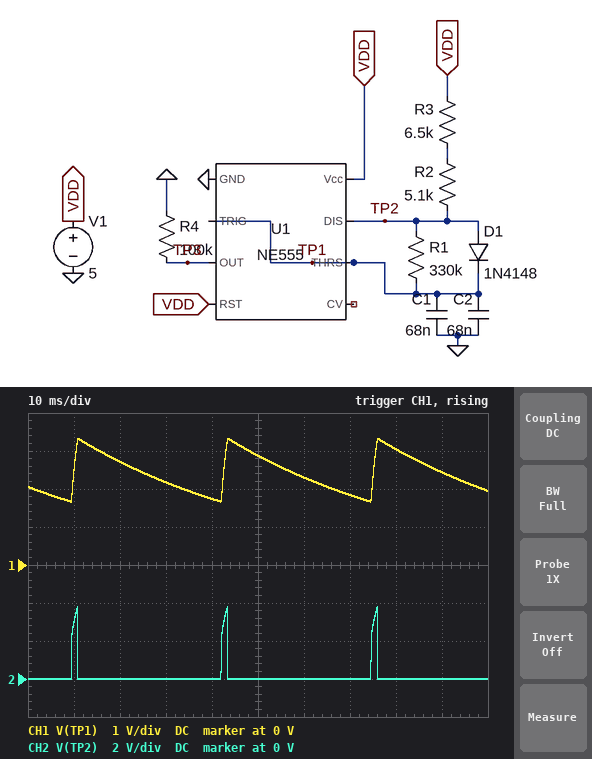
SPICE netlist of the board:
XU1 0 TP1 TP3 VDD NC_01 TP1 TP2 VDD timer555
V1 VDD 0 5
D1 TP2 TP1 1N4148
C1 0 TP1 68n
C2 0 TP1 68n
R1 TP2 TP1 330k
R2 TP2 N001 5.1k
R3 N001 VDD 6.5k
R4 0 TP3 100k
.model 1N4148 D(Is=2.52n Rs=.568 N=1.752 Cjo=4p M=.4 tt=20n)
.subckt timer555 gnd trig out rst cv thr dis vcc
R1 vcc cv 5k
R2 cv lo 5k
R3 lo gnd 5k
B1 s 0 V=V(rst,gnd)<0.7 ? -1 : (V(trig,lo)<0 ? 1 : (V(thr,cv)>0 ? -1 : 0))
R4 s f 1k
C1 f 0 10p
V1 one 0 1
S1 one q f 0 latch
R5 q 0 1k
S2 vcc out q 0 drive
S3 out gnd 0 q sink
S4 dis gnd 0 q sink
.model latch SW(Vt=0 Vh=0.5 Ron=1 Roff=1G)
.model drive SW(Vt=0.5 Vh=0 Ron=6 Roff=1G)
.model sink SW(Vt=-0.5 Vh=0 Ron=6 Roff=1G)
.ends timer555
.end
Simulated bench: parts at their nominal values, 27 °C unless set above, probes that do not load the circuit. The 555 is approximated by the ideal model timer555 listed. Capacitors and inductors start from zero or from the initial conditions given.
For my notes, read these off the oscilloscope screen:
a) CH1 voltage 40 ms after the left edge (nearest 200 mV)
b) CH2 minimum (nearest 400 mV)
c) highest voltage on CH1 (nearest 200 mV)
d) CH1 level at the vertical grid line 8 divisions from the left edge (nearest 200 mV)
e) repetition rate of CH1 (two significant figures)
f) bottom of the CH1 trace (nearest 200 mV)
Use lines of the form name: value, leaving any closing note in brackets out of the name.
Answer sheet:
CH1 voltage 40 ms after the left edge: 1.8 V
CH2 minimum: 0 V
highest voltage on CH1: 3.4 V
CH1 level at the vertical grid line 8 divisions from the left edge: 3.0 V
repetition rate of CH1: 31 Hz
bottom of the CH1 trace: 1.6 V
